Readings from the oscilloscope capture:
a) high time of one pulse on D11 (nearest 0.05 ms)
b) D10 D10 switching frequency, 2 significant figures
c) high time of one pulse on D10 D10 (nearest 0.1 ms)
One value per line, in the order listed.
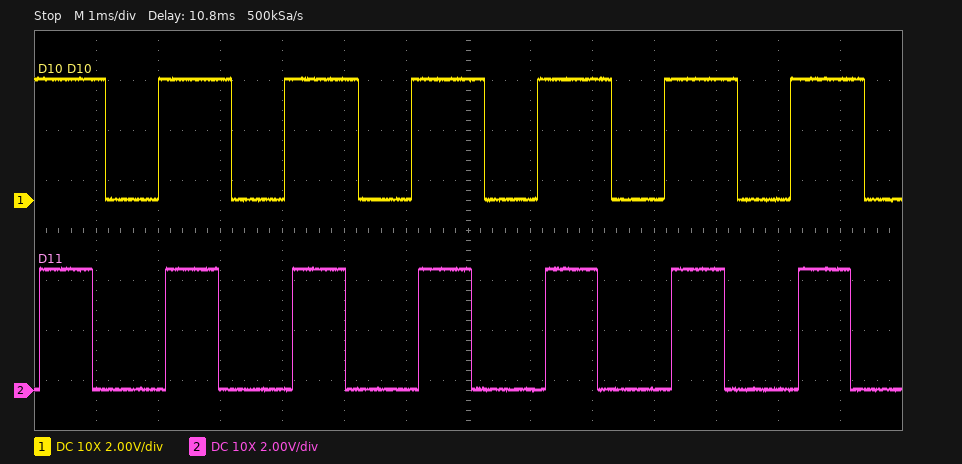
0.85 ms
490 Hz
1.2 ms
